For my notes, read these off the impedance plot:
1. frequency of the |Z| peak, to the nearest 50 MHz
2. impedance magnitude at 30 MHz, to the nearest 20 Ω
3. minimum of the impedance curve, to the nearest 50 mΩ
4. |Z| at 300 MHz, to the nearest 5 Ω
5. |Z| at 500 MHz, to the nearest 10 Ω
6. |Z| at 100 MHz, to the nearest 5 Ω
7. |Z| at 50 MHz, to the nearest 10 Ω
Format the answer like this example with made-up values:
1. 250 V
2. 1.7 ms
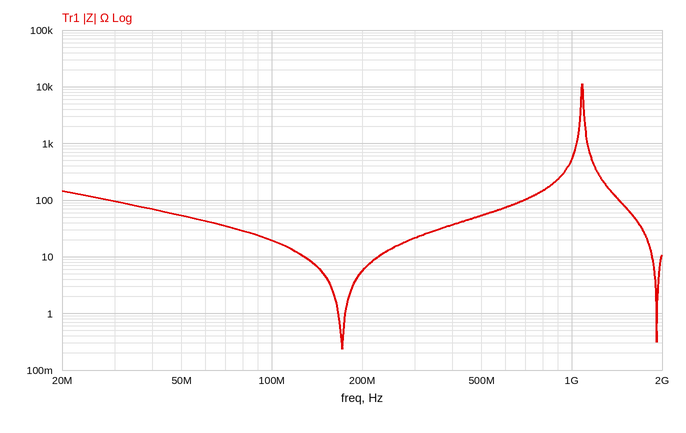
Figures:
1. 1.10 GHz
2. 100 Ω
3. 250 mΩ
4. 20 Ω
5. 50 Ω
6. 20 Ω
7. 50 Ω
